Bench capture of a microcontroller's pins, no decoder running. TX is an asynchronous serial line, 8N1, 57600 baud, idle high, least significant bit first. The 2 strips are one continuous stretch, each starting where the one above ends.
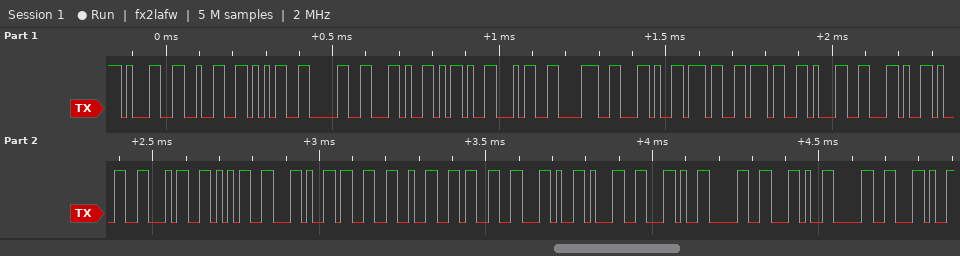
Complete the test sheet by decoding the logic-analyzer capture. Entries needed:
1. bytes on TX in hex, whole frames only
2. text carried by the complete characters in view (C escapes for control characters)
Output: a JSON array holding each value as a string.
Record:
["31 32 35 30 2C 2D 34 38 2C 37 37 31 2C 31 34 35 2C 33 32 33 2C 31 2C 30 2C 30 2C", "\"1250,-48,771,145,323,1,0,0,\""]
